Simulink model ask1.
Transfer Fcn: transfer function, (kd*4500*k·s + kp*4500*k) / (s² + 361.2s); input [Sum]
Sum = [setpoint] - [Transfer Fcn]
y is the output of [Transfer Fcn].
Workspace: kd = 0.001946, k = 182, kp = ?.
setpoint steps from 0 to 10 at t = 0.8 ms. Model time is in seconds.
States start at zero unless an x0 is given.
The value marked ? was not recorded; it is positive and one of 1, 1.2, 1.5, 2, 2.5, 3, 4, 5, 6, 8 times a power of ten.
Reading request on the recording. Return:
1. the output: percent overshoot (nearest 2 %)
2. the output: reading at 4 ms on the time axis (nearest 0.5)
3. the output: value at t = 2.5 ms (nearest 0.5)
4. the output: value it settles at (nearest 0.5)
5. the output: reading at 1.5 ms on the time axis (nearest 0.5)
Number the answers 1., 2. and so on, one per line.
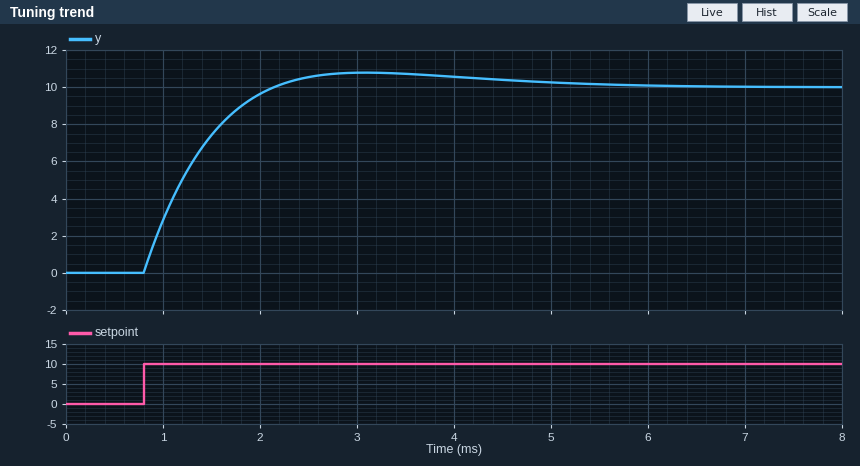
1. 8 %
2. 10.5
3. 10.5
4. 10.0
5. 7.5
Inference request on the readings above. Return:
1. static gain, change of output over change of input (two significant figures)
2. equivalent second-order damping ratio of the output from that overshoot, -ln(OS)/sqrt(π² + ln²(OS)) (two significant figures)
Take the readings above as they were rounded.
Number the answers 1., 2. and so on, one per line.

1. 1.0
2. 0.63
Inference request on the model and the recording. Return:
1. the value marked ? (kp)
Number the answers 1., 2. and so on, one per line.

1. 1.5
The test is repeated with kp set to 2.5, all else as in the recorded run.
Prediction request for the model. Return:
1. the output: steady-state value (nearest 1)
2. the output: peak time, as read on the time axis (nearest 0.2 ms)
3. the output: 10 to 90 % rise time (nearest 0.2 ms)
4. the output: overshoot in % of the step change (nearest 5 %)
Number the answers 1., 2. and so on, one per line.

1. 10
2. 2.6 ms
3. 0.8 ms
4. 15 %
